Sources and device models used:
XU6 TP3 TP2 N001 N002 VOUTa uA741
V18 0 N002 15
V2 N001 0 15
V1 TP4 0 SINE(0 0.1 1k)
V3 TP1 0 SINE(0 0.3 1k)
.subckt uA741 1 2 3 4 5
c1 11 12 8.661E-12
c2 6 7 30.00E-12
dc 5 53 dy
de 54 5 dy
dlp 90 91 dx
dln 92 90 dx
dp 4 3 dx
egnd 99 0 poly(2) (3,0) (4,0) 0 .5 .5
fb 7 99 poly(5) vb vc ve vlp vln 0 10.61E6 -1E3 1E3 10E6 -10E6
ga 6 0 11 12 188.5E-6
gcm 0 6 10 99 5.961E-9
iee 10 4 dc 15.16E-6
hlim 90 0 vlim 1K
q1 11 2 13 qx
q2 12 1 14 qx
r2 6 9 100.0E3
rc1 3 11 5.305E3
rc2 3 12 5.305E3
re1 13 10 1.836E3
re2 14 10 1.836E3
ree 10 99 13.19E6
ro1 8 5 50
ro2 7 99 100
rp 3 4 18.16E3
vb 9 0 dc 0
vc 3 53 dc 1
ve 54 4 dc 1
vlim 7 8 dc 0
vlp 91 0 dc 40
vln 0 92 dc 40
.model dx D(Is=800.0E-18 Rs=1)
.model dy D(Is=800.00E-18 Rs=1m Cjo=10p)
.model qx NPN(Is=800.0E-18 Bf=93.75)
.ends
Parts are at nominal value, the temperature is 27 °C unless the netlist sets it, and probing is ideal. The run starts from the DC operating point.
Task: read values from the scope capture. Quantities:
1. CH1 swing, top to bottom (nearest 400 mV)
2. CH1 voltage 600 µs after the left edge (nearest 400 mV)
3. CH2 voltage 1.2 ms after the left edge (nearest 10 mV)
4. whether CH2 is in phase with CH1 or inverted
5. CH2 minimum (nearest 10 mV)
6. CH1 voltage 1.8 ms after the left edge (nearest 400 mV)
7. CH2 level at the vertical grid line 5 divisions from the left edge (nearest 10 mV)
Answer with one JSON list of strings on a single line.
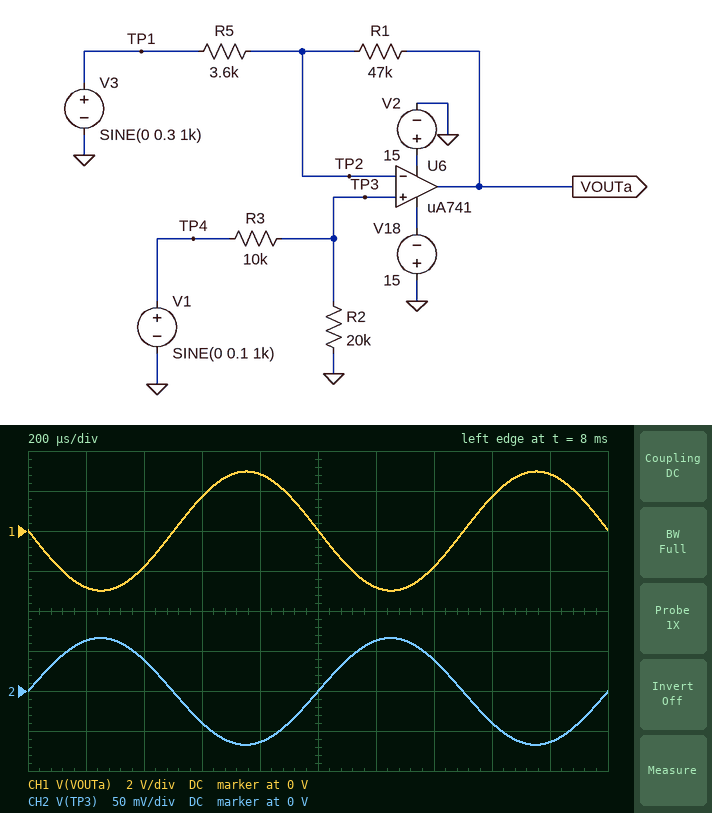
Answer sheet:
["6.0 V", "1.6 V", "60 mV", "inverted", "-70 mV", "2.8 V", "0 V"]
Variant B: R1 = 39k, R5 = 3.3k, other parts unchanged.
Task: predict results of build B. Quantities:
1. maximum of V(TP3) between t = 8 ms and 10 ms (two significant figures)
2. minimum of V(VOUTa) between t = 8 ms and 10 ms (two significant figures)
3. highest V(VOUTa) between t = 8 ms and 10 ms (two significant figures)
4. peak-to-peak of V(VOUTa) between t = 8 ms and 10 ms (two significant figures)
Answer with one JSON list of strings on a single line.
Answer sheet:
["66 mV", "-2.7 V", "2.7 V", "5.4 V"]
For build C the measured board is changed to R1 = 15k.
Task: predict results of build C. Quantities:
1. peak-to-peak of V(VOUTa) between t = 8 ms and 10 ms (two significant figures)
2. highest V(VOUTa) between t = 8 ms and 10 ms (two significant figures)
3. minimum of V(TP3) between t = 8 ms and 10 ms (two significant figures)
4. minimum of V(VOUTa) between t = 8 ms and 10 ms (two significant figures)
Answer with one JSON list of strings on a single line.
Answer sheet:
["1.8 V", "900 mV", "-67 mV", "-910 mV"]
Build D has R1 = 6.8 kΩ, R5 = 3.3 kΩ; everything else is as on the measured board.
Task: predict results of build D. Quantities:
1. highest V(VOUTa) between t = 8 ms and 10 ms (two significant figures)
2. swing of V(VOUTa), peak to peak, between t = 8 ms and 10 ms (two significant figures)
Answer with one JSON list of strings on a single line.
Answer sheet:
["410 mV", "830 mV"]
